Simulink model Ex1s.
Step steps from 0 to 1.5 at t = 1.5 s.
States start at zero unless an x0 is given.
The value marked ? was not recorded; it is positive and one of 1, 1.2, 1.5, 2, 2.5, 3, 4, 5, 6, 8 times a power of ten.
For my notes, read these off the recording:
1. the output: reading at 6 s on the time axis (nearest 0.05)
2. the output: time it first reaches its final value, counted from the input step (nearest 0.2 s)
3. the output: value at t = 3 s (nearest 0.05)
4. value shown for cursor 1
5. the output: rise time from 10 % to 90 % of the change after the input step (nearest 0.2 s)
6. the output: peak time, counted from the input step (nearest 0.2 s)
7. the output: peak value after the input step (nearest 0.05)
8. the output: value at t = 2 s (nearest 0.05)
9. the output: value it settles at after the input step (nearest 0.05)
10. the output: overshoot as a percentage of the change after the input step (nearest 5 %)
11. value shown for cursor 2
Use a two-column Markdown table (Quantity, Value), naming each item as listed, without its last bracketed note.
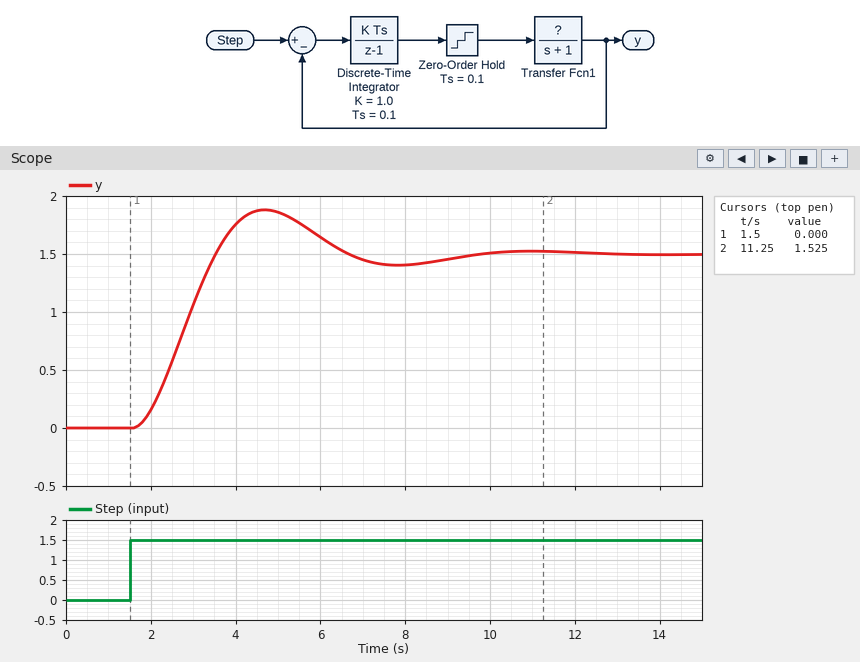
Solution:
| Quantity | Value |
|---|---|
| the output: reading at 6 s on the time axis | 1.65 |
| the output: time it first reaches its final value, counted from the input step | 2.0 s |
| the output: value at t = 3 s | 1.05 |
| value shown for cursor 1 | 0.000 |
| the output: rise time from 10 % to 90 % of the change after the input step | 1.4 s |
| the output: peak time, counted from the input step | 3.2 s |
| the output: peak value after the input step | 1.90 |
| the output: value at t = 2 s | 0.15 |
| the output: value it settles at after the input step | 1.50 |
| the output: overshoot as a percentage of the change after the input step | 25 % |
| value shown for cursor 2 | 1.525 |
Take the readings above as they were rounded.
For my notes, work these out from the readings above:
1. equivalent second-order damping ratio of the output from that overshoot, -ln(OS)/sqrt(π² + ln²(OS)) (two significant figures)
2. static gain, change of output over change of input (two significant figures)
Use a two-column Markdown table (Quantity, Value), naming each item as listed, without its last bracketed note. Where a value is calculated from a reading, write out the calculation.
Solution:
| Quantity | Value |
|---|---|
| equivalent second-order damping ratio of the output from that overshoot, -ln(OS)/sqrt(π² + ln²(OS)) | ln(0.25) = -1.386; 1.386 / sqrt(9.870 + 1.922) = 0.40 |
| static gain, change of output over change of input | (1.5 - 0) / (1.5 - 0) = 1.0 |
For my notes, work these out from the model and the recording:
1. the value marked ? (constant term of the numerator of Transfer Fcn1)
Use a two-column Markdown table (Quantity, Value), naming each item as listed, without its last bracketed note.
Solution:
| Quantity | Value |
|---|---|
| the value marked ? | 1.2 |
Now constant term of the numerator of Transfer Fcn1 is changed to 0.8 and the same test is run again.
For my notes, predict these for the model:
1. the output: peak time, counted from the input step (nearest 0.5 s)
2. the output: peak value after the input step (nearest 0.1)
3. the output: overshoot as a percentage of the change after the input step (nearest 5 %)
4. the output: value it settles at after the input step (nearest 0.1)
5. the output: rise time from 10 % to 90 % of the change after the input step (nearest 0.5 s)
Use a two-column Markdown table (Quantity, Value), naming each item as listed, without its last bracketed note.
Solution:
| Quantity | Value |
|---|---|
| the output: peak time, counted from the input step | 4.0 s |
| the output: peak value after the input step | 1.7 |
| the output: overshoot as a percentage of the change after the input step | 15 % |
| the output: value it settles at after the input step | 1.5 |
| the output: rise time from 10 % to 90 % of the change after the input step | 2.0 s |
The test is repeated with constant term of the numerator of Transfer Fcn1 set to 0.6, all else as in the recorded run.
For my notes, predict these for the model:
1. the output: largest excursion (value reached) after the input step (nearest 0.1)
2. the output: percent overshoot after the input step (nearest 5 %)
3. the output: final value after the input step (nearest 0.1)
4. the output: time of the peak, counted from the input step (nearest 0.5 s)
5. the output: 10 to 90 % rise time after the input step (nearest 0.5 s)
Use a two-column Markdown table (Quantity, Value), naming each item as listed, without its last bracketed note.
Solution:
| Quantity | Value |
|---|---|
| the output: largest excursion (value reached) after the input step | 1.6 |
| the output: percent overshoot after the input step | 10 % |
| the output: final value after the input step | 1.5 |
| the output: time of the peak, counted from the input step | 5.0 s |
| the output: 10 to 90 % rise time after the input step | 2.5 s |
